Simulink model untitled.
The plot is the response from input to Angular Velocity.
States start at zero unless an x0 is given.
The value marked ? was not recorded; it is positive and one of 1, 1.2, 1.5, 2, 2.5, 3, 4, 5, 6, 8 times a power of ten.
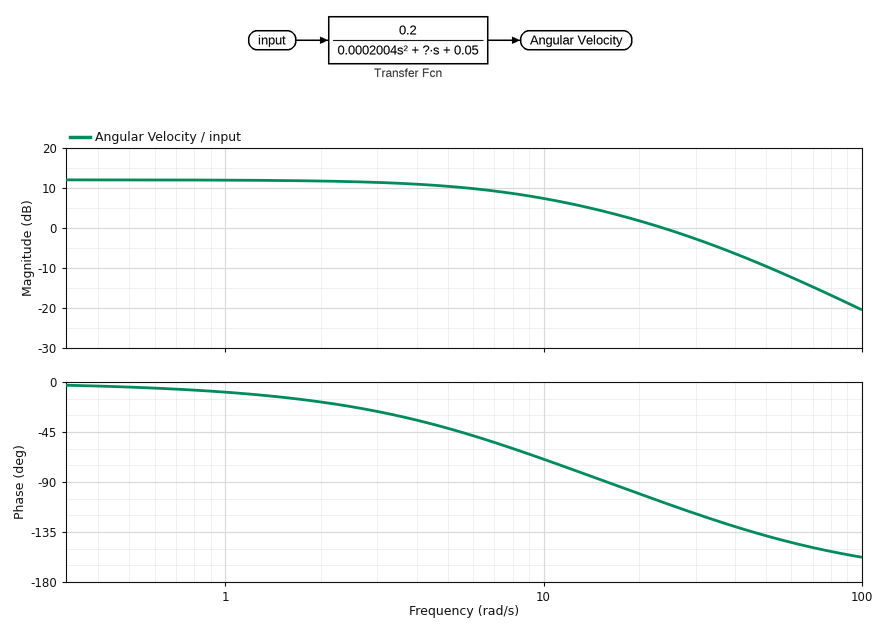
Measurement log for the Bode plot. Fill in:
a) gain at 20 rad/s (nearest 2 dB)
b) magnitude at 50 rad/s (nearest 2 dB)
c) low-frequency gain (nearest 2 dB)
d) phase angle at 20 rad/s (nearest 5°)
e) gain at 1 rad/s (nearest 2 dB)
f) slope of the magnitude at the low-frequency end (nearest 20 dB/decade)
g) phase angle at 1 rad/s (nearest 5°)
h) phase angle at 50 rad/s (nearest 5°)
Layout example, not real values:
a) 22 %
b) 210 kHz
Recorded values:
a) 2 dB
b) -10 dB
c) 12 dB
d) -100°
e) 12 dB
f) 0 dB/decade
g) -10°
h) -140°
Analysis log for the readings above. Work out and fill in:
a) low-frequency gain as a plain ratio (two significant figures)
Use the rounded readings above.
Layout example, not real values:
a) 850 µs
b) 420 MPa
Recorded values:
a) 4.0
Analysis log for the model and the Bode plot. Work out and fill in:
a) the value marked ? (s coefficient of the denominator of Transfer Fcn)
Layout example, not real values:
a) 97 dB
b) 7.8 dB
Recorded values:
a) 0.008
